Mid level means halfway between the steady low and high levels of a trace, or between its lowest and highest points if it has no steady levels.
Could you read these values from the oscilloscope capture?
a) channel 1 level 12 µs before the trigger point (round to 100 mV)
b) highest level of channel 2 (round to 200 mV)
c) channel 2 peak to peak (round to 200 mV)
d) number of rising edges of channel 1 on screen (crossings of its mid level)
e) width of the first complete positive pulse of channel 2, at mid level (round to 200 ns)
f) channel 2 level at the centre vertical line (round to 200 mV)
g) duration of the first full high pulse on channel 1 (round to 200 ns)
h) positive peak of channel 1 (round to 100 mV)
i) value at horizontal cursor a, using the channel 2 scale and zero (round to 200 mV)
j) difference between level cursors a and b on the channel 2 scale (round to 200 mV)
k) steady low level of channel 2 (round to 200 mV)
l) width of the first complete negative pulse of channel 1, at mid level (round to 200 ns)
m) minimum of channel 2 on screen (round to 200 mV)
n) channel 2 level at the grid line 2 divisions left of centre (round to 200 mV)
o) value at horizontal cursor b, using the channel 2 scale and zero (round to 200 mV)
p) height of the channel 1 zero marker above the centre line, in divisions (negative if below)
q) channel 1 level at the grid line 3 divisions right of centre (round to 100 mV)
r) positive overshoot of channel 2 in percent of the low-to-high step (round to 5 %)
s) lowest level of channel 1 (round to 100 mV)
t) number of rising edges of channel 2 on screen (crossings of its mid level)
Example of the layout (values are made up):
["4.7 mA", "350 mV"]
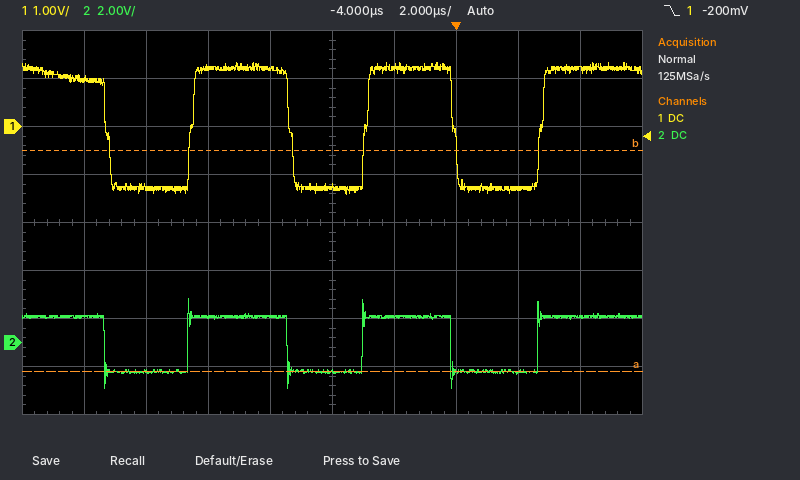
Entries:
["1.0 V", "1.8 V", "3.8 V", "3", "3.2 µs", "-1.2 V", "3.2 µs", "1.3 V", "-1.2 V", "9.2 V", "-1.2 V", "2.8 µs", "-2.0 V", "1.0 V", "8.0 V", "+2.0 div", "-1.3 V", "30 %", "-1.4 V", "3"]
